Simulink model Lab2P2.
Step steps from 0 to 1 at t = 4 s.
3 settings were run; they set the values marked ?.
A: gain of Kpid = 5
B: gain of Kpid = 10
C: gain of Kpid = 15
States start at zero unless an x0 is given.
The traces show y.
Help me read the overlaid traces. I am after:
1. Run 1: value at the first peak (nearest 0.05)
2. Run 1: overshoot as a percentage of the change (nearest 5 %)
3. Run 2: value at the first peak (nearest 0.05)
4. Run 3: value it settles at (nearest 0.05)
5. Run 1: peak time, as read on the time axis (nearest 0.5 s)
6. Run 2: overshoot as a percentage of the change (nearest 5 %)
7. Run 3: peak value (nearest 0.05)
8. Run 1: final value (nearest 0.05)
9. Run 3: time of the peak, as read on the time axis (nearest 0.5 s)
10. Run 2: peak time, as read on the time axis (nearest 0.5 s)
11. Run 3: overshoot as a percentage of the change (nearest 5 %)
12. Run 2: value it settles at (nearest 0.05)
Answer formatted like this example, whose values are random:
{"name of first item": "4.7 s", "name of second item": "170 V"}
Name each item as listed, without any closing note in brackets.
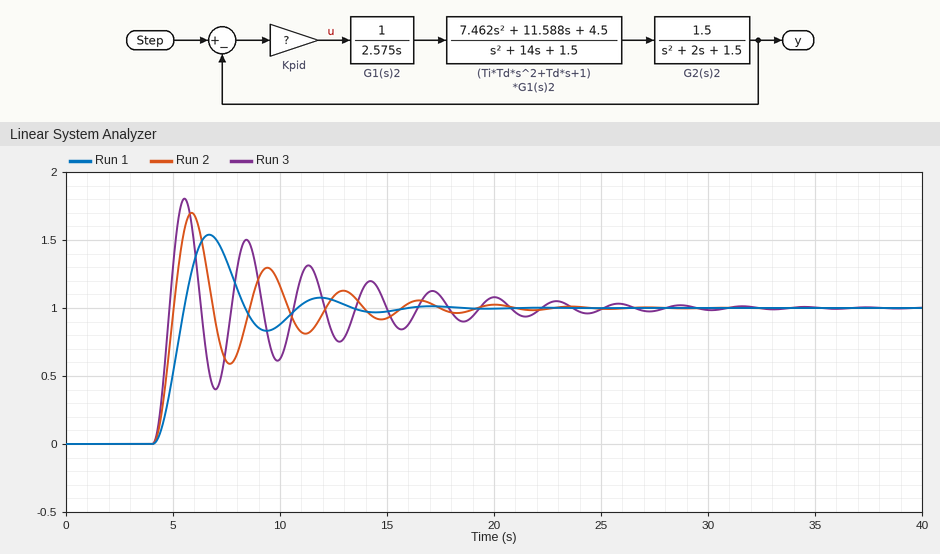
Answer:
{"Run 1: value at the first peak": "1.55", "Run 1: overshoot as a percentage of the change": "55 %", "Run 2: value at the first peak": "1.70", "Run 3: value it settles at": "1.00", "Run 1: peak time, as read on the time axis": "6.5 s", "Run 2: overshoot as a percentage of the change": "70 %", "Run 3: peak value": "1.80", "Run 1: final value": "1.00", "Run 3: time of the peak, as read on the time axis": "5.5 s", "Run 2: peak time, as read on the time axis": "6.0 s", "Run 3: overshoot as a percentage of the change": "80 %", "Run 2: value it settles at": "1.00"}
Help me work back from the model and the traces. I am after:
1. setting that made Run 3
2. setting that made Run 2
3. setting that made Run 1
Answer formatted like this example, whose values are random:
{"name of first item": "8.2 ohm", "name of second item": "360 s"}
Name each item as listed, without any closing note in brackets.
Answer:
{"setting that made Run 3": "C", "setting that made Run 2": "B", "setting that made Run 1": "A"}
